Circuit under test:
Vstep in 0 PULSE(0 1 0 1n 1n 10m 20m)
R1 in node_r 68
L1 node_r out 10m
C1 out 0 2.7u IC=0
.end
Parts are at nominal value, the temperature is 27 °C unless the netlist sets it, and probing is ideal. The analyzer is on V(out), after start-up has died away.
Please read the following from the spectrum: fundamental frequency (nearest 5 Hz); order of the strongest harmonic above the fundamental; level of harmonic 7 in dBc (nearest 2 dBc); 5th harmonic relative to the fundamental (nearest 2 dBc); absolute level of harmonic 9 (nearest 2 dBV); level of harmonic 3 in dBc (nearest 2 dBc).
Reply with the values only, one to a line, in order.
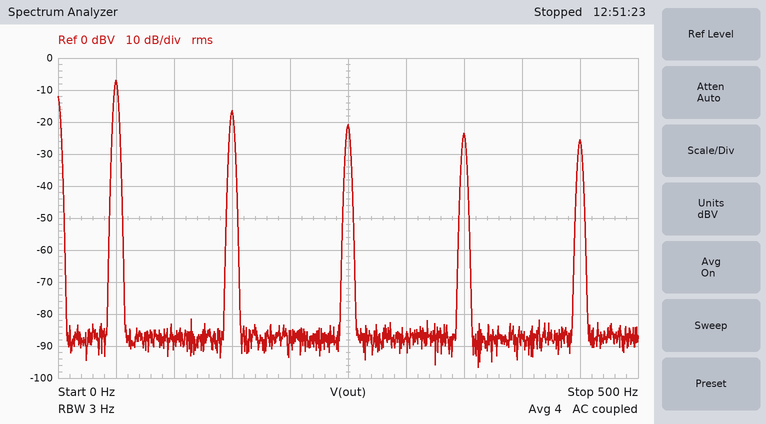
50 Hz
3
-16 dBc
-14 dBc
-26 dBV
-10 dBc
